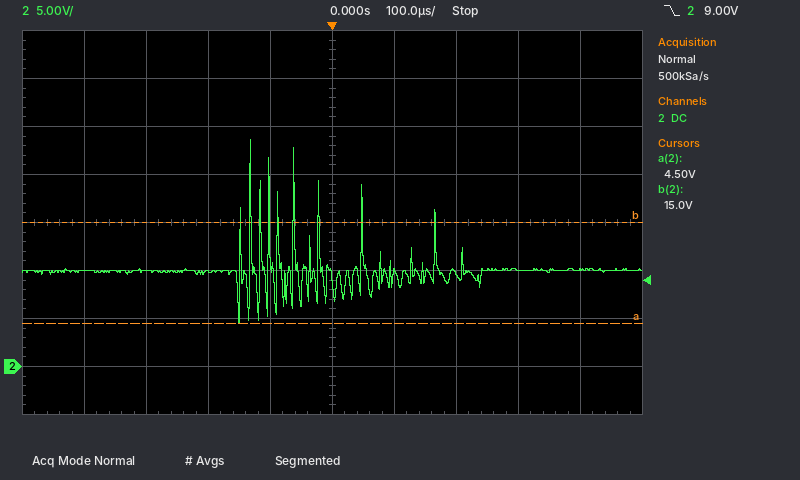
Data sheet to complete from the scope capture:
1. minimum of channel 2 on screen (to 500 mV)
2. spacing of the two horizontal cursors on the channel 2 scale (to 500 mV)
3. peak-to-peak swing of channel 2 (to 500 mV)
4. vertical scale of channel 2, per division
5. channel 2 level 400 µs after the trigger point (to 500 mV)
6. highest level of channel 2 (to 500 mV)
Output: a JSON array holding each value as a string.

["4.5 V", "10.5 V", "19.0 V", "5 V", "10.0 V", "23.5 V"]
